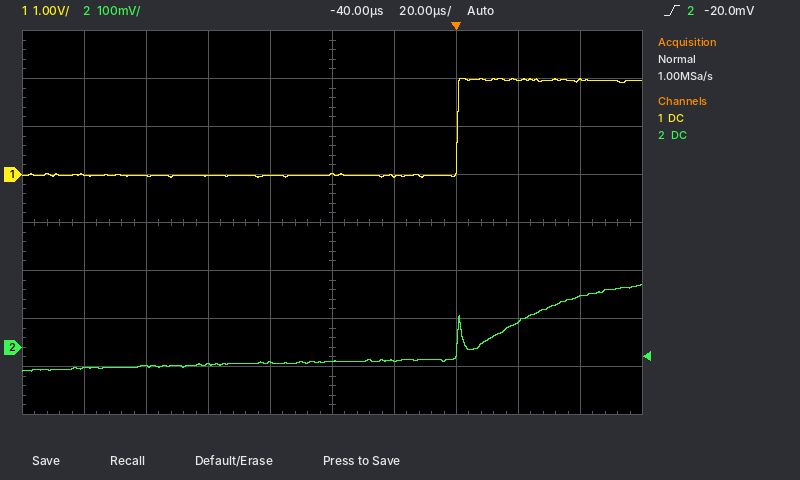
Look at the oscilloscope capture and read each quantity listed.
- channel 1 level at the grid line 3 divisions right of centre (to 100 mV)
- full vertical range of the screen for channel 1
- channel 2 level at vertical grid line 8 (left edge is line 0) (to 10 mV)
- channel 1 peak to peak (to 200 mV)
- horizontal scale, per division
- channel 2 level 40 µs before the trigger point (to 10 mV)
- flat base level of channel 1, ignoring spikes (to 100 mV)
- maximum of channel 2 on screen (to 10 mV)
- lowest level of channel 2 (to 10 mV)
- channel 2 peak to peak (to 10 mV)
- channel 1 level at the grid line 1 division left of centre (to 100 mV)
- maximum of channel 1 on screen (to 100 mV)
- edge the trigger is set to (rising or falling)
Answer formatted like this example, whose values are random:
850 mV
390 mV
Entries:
2.0 V
8 V
50 mV
2.0 V
20 µs
-30 mV
0.0 V
130 mV
-50 mV
180 mV
0.0 V
2.0 V
rising
